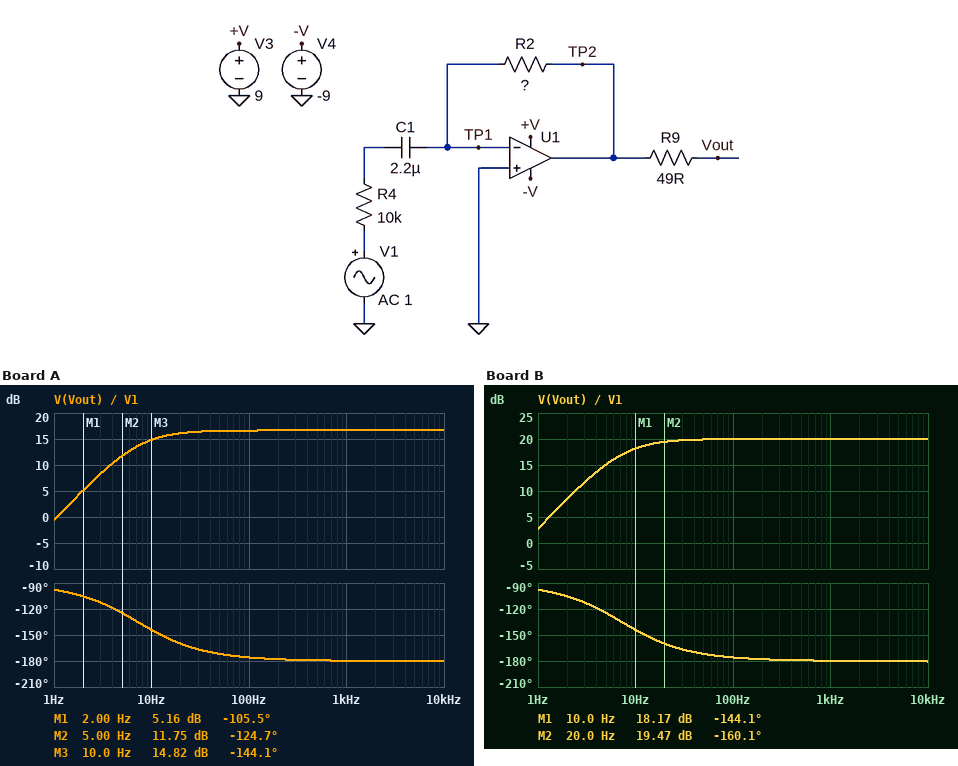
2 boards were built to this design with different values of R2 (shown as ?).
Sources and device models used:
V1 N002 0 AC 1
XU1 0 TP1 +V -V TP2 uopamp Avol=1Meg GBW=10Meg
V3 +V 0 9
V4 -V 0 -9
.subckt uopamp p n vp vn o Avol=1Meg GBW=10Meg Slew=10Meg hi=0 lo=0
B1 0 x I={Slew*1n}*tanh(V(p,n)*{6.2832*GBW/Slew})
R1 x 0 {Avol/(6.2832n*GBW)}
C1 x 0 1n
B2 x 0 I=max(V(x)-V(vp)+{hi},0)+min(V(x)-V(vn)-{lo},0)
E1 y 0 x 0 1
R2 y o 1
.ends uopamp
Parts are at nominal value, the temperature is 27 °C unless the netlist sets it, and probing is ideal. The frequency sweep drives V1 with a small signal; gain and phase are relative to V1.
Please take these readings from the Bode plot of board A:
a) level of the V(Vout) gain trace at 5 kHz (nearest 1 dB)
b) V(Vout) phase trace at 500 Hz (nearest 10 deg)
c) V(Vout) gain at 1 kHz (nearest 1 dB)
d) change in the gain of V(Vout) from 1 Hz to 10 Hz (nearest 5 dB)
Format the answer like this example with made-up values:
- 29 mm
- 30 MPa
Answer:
- 17 dB
- -180 deg
- 17 dB
- 15 dB
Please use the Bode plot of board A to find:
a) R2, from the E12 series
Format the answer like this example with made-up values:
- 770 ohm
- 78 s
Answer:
- 68 kΩ
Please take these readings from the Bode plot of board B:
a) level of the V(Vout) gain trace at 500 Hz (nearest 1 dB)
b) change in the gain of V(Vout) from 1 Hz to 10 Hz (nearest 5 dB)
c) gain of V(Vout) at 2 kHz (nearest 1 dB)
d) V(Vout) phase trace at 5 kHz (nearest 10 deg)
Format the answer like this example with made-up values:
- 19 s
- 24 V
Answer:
- 20 dB
- 15 dB
- 20 dB
- -180 deg
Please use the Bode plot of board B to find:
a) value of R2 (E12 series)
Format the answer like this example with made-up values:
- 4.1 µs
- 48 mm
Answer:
- 100 kΩ
